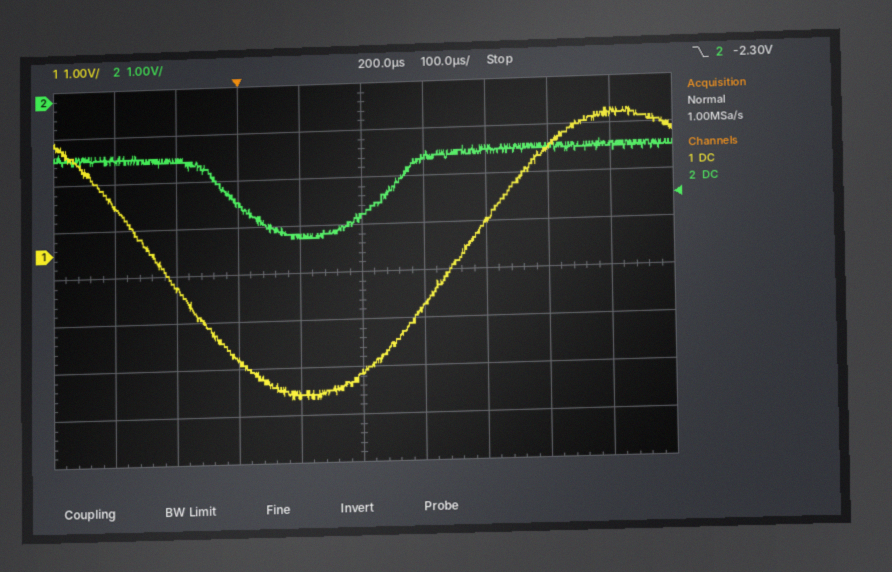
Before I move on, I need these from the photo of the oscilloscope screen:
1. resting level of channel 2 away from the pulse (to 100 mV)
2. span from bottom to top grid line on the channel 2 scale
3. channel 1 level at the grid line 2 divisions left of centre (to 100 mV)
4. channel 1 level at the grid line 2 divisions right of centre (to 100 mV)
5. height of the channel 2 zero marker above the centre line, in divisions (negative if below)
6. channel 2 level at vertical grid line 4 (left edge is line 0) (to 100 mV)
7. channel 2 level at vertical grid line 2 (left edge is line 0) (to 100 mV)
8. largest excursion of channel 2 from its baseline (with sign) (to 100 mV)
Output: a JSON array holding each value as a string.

["-1.3 V", "8 V", "-2.3 V", "500 mV", "+3.8 div", "-3.0 V", "-1.3 V", "-1.8 V"]
